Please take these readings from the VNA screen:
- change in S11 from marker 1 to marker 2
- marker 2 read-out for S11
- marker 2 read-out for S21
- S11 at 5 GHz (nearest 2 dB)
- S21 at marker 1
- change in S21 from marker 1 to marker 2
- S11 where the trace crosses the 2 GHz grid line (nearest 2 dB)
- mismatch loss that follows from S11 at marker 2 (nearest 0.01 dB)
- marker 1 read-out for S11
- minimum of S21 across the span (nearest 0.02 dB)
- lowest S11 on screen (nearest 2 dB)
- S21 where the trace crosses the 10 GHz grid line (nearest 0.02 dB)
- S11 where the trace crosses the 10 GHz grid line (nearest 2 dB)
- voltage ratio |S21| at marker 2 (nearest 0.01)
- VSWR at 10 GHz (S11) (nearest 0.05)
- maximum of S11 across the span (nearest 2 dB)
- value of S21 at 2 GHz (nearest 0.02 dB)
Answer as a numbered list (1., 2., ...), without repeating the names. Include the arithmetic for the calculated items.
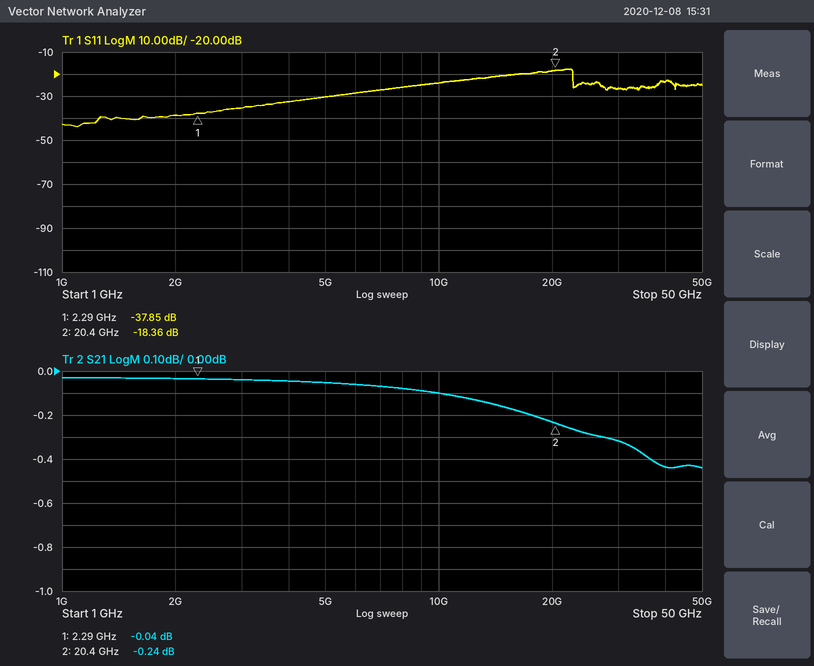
1. -18.36 − (-37.85) = 19.49 dB
2. -18.36 dB
3. -0.24 dB
4. -30 dB
5. -0.04 dB
6. -0.24 − (-0.04) = -0.20 dB
7. -38 dB
8. −10 log10(1 − 10^(-18.36/10)) ≈ 0.06 dB
9. -37.85 dB
10. -0.44 dB
11. -44 dB
12. -0.10 dB
13. -24 dB
14. 10^(-0.24/20) ≈ 0.97
15. |Γ| = 10^(-24/20) = 0.0631; VSWR = (1 + 0.0631)/(1 − 0.0631) ≈ 1.13, so 1.15 to the nearest 0.05
16. -18 dB
17. -0.04 dB
